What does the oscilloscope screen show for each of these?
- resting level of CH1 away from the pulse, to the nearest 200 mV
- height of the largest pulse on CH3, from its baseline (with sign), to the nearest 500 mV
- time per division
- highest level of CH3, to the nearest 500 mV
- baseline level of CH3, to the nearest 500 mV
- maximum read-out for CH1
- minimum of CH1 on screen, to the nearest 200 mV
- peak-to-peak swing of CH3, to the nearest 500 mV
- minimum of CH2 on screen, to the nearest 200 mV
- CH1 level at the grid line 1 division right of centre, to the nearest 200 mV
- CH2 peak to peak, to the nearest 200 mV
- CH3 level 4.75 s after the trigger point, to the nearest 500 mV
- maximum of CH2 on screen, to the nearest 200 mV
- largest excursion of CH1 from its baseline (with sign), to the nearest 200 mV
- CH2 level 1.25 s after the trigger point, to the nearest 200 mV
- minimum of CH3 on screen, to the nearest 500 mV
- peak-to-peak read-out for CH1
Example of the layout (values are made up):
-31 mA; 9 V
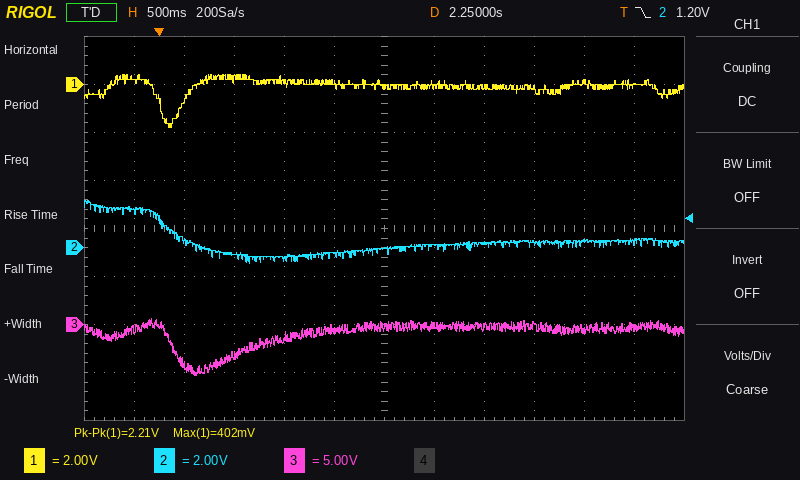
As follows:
0.0 V; -5.0 V; 500 ms; 500 mV; -500 mV; 402 mV; -1.8 V; 6.0 V; -600 mV; 0.0 V; 2.6 V; -500 mV; 2.0 V; -1.8 V; -400 mV; -5.5 V; 2.21 V
